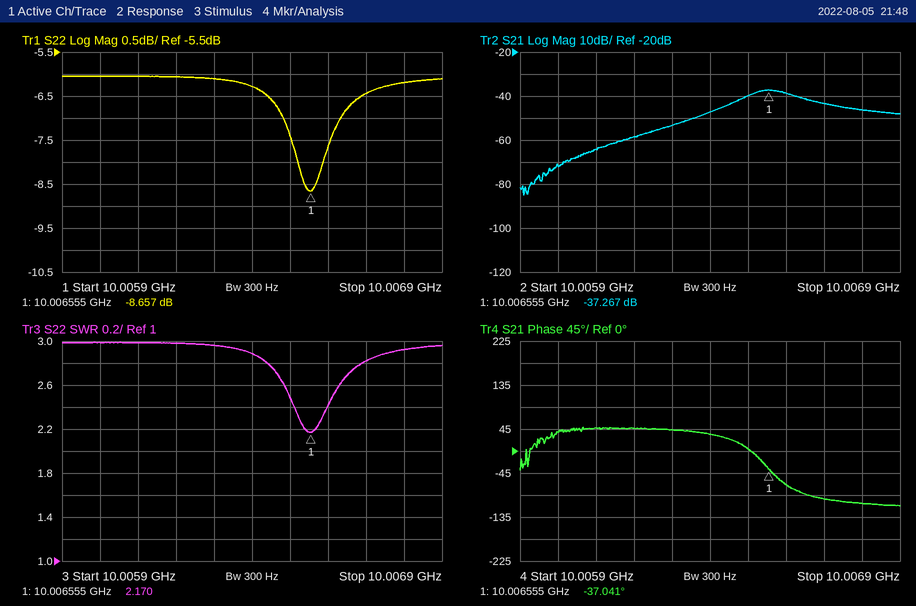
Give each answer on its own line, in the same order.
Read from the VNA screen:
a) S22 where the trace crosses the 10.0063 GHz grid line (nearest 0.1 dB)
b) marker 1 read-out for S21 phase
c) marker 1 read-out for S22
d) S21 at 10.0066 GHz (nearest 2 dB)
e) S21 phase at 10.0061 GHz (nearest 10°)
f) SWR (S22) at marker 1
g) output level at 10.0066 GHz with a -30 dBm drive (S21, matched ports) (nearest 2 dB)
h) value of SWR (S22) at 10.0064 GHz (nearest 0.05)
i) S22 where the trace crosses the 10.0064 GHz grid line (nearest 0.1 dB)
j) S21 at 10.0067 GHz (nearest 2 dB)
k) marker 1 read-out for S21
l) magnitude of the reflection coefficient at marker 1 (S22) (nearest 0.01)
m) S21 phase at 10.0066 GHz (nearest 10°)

-6.1 dB
-37.041°
-8.657 dB
-38 dB
50°
2.170
-68 dBm
2.90
-6.3 dB
-44 dB
-37.267 dB
0.37
-70°
